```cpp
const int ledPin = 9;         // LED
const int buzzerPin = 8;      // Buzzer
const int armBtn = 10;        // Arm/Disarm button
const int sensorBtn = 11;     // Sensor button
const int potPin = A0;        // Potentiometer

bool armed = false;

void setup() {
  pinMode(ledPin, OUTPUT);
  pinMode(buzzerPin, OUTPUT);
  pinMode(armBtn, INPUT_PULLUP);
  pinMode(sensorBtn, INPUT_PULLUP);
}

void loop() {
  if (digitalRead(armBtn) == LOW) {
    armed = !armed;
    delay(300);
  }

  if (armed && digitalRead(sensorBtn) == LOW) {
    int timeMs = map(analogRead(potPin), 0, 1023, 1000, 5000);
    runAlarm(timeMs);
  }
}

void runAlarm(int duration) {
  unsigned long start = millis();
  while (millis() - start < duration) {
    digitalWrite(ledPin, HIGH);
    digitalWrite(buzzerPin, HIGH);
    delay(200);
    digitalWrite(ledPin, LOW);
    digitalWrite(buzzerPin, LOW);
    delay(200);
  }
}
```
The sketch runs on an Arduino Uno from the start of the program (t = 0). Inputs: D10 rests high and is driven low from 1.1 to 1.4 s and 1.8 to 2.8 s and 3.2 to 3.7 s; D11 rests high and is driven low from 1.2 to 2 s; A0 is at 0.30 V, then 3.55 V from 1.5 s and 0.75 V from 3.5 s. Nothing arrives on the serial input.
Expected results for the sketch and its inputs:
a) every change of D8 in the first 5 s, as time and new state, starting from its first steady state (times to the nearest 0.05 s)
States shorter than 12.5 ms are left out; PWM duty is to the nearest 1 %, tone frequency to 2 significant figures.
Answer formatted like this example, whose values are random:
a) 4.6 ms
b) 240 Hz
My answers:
a) 0 s low; 1.4 s high; 1.6 s low; 1.8 s high; 2 s low; 2.2 s high; 2.4 s low; 2.6 s high; 2.8 s low
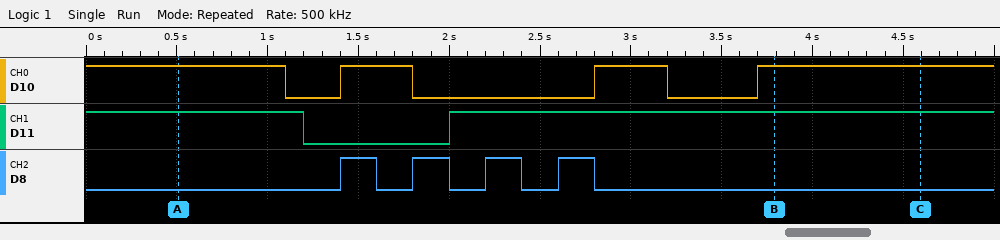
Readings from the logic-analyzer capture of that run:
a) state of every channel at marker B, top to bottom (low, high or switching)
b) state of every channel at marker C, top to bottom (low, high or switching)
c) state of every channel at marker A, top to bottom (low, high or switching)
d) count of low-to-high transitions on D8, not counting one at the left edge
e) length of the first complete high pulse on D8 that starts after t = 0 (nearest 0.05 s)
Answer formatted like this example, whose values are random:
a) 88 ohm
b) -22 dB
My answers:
a) D10 high, D11 high, D8 low
b) D10 high, D11 high, D8 low
c) D10 high, D11 high, D8 low
d) 4
e) 0.20 s
